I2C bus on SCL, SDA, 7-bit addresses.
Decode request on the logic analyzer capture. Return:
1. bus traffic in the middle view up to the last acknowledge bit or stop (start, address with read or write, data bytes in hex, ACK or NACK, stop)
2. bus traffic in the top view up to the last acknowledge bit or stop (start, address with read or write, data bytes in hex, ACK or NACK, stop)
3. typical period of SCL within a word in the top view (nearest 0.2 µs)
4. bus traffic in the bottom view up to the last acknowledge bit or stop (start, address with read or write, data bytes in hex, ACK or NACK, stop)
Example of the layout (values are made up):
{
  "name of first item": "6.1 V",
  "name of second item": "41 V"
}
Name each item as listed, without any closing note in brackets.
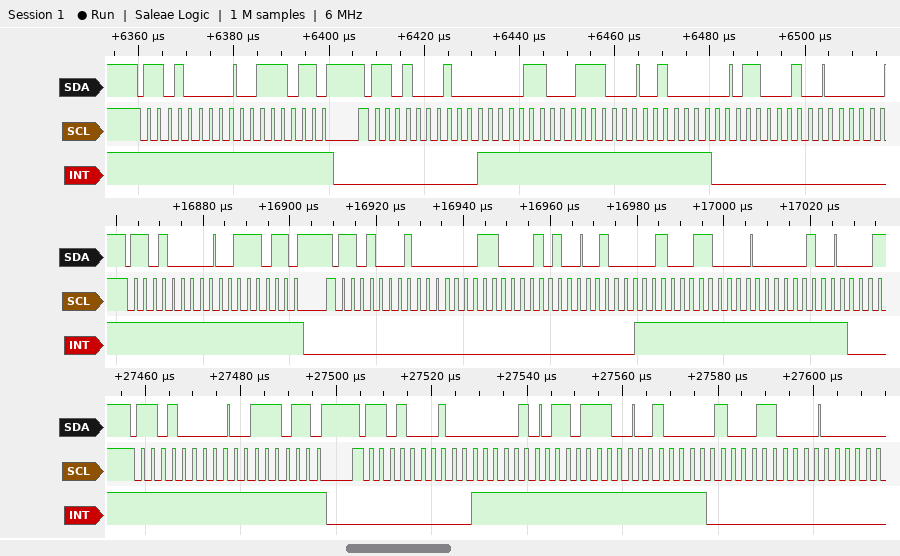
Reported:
{
  "bus traffic in the middle view up to the last acknowledge bit or stop": "start, address 68 write ACK, 3B ACK, repeated start, address 68 read ACK, 03 ACK, 14 ACK, 41 ACK, 30 ACK, 04 ACK",
  "bus traffic in the top view up to the last acknowledge bit or stop": "start, address 68 write ACK, 3B ACK, repeated start, address 68 read ACK, 03 ACK, 38 ACK, 40 ACK, C4 ACK",
  "typical period of SCL within a word in the top view": "2.2 µs",
  "bus traffic in the bottom view up to the last acknowledge bit or stop": "start, address 68 write ACK, 3B ACK, repeated start, address 68 read ACK, 02 ACK, DC ACK, 41 ACK, 30 ACK"
}
